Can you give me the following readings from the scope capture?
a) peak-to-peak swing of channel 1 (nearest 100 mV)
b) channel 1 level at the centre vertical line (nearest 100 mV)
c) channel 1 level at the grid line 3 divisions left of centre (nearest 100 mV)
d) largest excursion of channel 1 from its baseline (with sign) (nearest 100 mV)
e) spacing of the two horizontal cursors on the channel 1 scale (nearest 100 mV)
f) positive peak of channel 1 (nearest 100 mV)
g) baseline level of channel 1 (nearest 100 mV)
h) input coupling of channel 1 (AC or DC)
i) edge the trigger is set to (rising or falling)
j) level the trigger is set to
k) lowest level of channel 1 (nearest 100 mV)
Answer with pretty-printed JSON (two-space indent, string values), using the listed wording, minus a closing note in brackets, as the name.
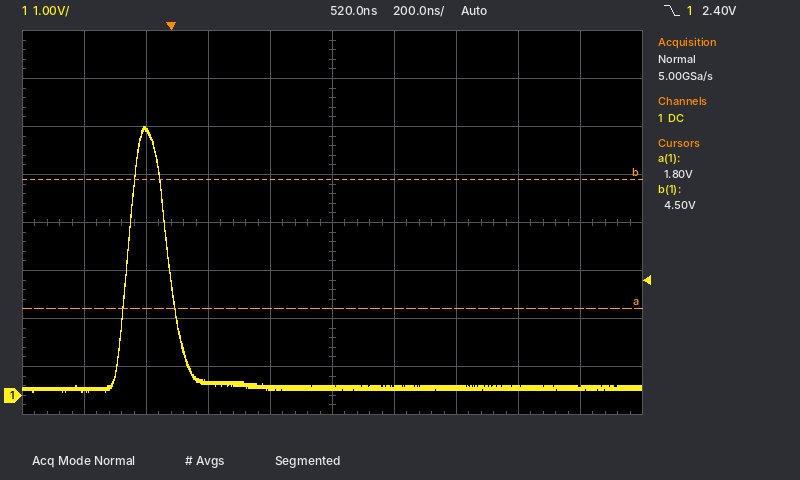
{
  "peak-to-peak swing of channel 1": "5.5 V",
  "channel 1 level at the centre vertical line": "200 mV",
  "channel 1 level at the grid line 3 divisions left of centre": "5.5 V",
  "largest excursion of channel 1 from its baseline (with sign)": "+5.4 V",
  "spacing of the two horizontal cursors on the channel 1 scale": "2.7 V",
  "positive peak of channel 1": "5.6 V",
  "baseline level of channel 1": "200 mV",
  "input coupling of channel 1": "DC",
  "edge the trigger is set to": "falling",
  "level the trigger is set to": "2.40 V",
  "lowest level of channel 1": "100 mV"
}
